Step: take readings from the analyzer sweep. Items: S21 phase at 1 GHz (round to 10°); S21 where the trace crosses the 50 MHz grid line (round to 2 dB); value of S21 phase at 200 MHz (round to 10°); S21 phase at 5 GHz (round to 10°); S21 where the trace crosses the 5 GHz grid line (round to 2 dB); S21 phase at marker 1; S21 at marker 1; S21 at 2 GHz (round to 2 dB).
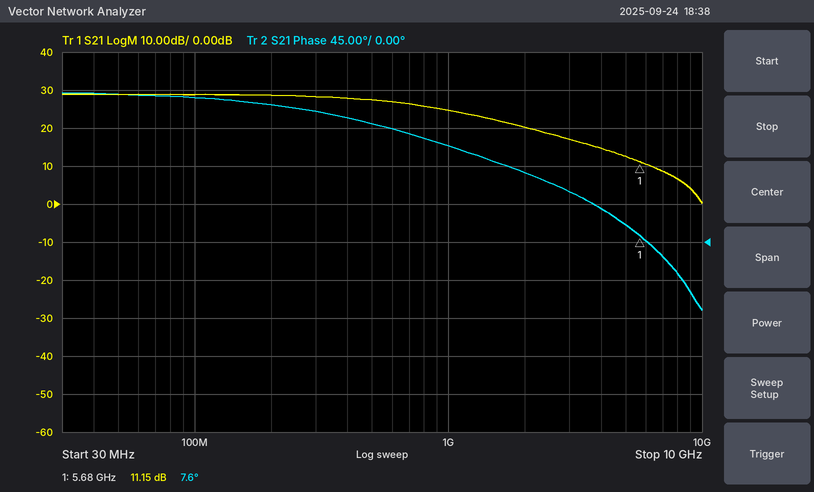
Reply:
110°
28 dB
160°
20°
12 dB
7.6°
11.15 dB
20 dB
